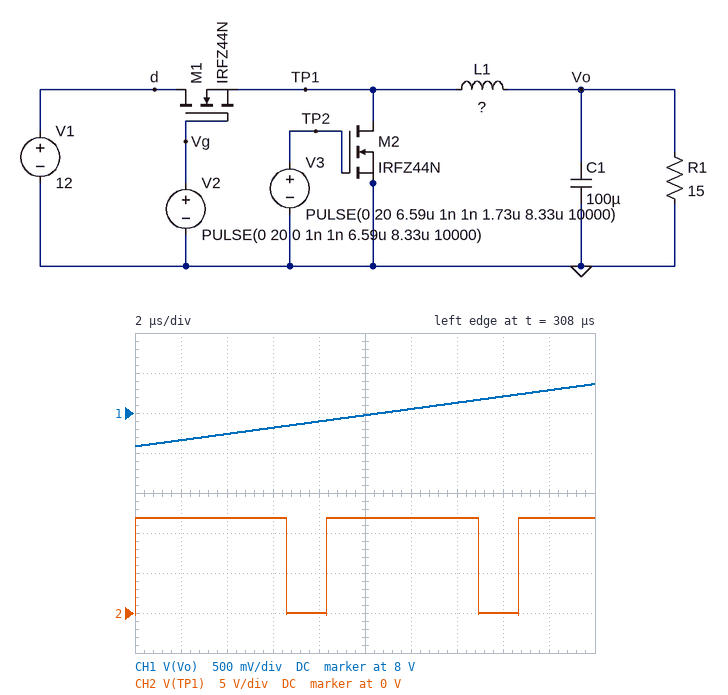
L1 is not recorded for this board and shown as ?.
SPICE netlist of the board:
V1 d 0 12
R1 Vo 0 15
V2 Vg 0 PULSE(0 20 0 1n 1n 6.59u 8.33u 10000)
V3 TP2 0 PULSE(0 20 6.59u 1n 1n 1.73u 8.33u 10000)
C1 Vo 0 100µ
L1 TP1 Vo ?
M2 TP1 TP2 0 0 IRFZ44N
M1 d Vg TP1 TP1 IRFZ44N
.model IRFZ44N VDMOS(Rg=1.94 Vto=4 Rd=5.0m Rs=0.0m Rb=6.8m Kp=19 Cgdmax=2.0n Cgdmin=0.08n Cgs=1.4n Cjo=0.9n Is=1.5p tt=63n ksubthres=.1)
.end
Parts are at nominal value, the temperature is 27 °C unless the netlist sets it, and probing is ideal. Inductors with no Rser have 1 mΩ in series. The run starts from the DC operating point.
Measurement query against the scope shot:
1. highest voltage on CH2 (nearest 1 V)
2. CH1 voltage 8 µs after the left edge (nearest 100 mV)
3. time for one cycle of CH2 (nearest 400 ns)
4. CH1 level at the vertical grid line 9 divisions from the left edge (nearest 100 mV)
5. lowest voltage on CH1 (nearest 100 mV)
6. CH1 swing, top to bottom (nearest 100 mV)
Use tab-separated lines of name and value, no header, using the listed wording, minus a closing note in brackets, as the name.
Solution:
highest voltage on CH2	12 V
CH1 voltage 8 µs after the left edge	7.9 V
time for one cycle of CH2	8.4 µs
CH1 level at the vertical grid line 9 divisions from the left edge	8.3 V
lowest voltage on CH1	7.6 V
CH1 swing, top to bottom	800 mV
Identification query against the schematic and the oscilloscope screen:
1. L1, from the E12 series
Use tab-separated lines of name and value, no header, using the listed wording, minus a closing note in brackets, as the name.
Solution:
L1, from the E12 series	470 µH
